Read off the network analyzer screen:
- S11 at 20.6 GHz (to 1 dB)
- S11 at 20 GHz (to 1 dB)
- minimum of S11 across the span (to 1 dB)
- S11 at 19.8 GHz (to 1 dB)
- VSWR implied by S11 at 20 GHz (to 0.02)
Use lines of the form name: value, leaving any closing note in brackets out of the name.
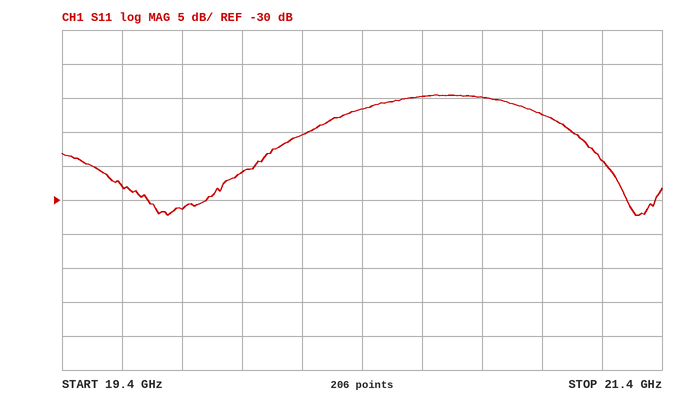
S11 at 20.6 GHz: -15 dB
S11 at 20 GHz: -26 dB
minimum of S11 across the span: -32 dB
S11 at 19.8 GHz: -31 dB
VSWR implied by S11 at 20 GHz: 1.10
